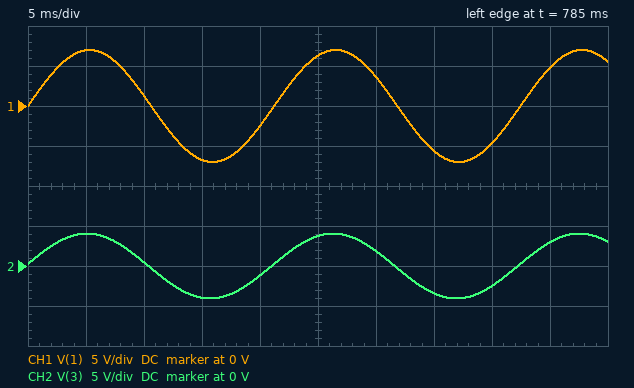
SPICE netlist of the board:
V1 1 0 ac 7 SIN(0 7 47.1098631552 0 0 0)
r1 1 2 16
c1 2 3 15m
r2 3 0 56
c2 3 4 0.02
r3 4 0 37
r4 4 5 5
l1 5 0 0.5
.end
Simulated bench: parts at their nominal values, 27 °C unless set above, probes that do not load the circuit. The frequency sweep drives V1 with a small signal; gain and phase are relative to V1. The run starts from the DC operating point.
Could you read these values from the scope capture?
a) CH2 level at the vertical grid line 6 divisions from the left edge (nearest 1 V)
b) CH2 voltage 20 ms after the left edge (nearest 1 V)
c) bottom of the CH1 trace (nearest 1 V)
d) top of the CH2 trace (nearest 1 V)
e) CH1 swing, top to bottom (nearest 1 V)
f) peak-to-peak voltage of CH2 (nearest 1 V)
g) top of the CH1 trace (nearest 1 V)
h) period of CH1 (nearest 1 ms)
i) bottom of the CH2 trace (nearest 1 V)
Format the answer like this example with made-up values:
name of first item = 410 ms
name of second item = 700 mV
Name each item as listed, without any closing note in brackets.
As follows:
CH2 level at the vertical grid line 6 divisions from the left edge = 2 V
CH2 voltage 20 ms after the left edge = -1 V
bottom of the CH1 trace = -7 V
top of the CH2 trace = 4 V
CH1 swing, top to bottom = 14 V
peak-to-peak voltage of CH2 = 8 V
top of the CH1 trace = 7 V
period of CH1 = 21 ms
bottom of the CH2 trace = -4 V
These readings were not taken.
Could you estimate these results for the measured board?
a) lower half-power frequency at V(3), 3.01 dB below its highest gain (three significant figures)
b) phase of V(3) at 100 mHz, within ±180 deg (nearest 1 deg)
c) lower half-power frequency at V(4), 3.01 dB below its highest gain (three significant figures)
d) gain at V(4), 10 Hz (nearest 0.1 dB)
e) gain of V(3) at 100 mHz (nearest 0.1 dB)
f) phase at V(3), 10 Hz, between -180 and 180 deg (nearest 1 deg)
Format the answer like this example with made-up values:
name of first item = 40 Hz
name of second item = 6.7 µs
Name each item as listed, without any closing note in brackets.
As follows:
lower half-power frequency at V(3), 3.01 dB below its highest gain = 4.56 Hz
phase of V(3) at 100 mHz, within ±180 deg = 34 deg
lower half-power frequency at V(4), 3.01 dB below its highest gain = 3.49 Hz
gain at V(4), 10 Hz = -5.2 dB
gain of V(3) at 100 mHz = -10.0 dB
phase at V(3), 10 Hz, between -180 and 180 deg = 17 deg
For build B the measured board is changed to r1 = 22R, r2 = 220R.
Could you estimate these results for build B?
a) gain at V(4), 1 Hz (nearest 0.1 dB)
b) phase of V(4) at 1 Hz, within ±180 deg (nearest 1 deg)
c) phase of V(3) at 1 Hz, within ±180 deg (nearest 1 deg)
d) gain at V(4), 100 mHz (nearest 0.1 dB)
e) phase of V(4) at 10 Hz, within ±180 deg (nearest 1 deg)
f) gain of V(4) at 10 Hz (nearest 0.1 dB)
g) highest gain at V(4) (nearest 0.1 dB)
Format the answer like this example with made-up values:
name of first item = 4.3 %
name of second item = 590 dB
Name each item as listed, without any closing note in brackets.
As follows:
gain at V(4), 1 Hz = -15.7 dB
phase of V(4) at 1 Hz, within ±180 deg = 60 deg
phase of V(3) at 1 Hz, within ±180 deg = -18 deg
gain at V(4), 100 mHz = -32.9 dB
phase of V(4) at 10 Hz, within ±180 deg = 23 deg
gain of V(4) at 10 Hz = -5.6 dB
highest gain at V(4) = -4.6 dB
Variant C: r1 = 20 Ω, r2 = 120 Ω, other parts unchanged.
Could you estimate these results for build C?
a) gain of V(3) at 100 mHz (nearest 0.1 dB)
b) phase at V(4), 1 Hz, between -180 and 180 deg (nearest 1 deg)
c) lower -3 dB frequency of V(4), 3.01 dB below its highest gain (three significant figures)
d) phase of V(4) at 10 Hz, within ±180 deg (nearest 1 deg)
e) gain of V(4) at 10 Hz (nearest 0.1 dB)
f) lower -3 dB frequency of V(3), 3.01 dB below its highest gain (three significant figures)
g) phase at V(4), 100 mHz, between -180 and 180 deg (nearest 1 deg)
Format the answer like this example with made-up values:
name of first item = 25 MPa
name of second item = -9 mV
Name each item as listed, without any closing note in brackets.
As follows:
gain of V(3) at 100 mHz = -8.3 dB
phase at V(4), 1 Hz, between -180 and 180 deg = 63 deg
lower -3 dB frequency of V(4), 3.01 dB below its highest gain = 4.42 Hz
phase of V(4) at 10 Hz, within ±180 deg = 22 deg
gain of V(4) at 10 Hz = -5.5 dB
lower -3 dB frequency of V(3), 3.01 dB below its highest gain = 5.36 Hz
phase at V(4), 100 mHz, between -180 and 180 deg = 106 deg
